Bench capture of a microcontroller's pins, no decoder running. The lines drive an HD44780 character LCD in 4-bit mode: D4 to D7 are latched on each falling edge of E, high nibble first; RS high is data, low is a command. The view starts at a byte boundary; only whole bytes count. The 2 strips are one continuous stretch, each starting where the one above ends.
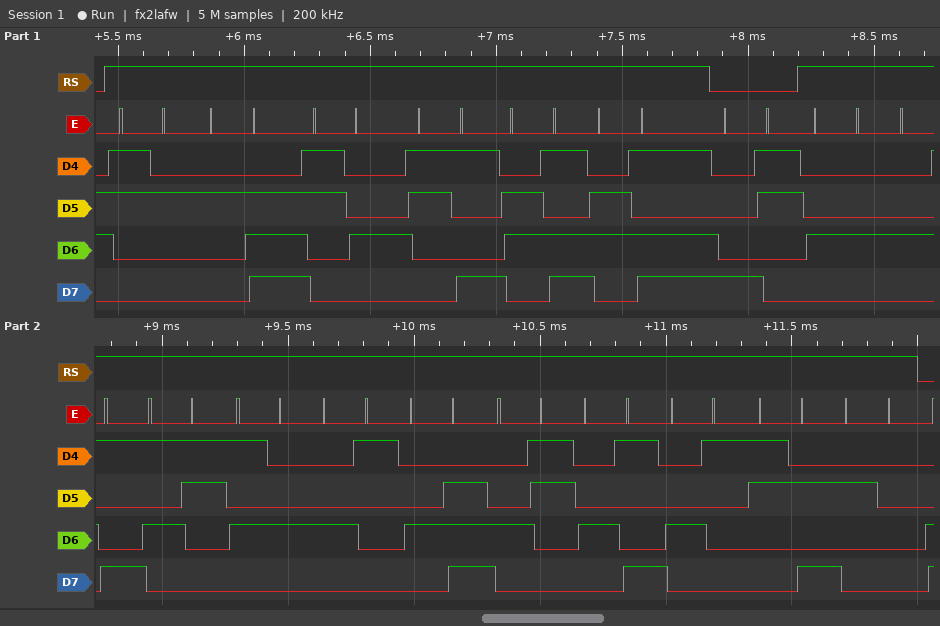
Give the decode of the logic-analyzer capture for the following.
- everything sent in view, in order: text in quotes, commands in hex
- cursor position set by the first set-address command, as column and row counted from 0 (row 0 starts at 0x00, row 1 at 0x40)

"2.49mm" 0x83 "DISTANCIA: "
column 3, row 0
